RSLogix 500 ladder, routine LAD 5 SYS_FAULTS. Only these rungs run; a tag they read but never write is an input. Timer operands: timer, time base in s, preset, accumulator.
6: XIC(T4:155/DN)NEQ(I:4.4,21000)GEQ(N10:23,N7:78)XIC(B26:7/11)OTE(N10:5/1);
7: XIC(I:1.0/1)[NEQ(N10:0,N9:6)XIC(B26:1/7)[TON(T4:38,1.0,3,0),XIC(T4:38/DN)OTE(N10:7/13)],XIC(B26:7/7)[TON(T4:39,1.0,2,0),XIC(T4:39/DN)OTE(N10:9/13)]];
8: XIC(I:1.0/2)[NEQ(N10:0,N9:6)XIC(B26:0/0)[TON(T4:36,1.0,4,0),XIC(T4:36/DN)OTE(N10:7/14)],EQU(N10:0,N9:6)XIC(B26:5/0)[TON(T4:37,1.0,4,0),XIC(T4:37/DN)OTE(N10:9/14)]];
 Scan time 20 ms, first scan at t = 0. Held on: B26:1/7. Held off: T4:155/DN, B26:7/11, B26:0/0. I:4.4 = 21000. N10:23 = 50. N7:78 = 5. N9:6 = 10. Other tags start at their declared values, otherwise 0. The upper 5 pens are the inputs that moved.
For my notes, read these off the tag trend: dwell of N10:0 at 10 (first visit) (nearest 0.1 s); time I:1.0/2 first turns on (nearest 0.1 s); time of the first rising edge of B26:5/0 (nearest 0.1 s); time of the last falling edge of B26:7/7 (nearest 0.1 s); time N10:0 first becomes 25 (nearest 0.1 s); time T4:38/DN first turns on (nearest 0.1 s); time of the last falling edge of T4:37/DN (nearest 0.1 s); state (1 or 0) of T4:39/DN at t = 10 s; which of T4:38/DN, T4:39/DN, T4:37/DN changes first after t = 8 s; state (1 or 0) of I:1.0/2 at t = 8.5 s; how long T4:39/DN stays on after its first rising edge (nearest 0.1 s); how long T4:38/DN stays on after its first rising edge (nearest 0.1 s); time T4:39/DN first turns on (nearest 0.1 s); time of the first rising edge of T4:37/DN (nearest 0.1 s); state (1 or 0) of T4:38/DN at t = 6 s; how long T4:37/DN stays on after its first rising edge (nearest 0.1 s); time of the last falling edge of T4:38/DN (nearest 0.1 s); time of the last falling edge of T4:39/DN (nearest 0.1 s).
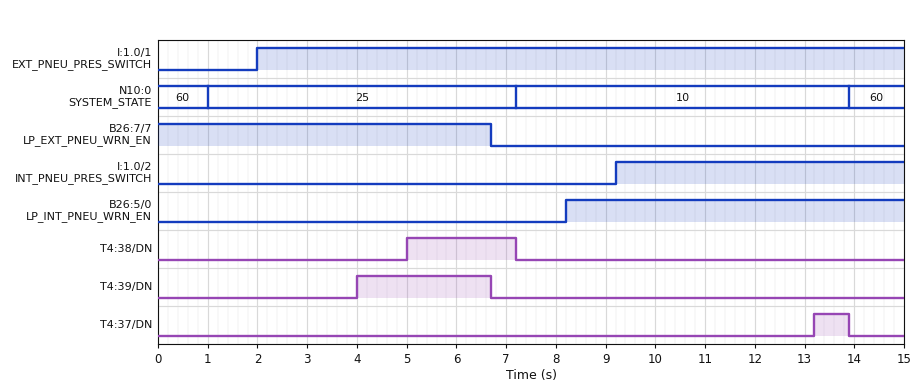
6.7 s
9.2 s
8.2 s
6.7 s
1.0 s
5.0 s
13.9 s
0
T4:37/DN
0
2.7 s
2.2 s
4.0 s
13.2 s
1
0.7 s
7.2 s
6.7 s
